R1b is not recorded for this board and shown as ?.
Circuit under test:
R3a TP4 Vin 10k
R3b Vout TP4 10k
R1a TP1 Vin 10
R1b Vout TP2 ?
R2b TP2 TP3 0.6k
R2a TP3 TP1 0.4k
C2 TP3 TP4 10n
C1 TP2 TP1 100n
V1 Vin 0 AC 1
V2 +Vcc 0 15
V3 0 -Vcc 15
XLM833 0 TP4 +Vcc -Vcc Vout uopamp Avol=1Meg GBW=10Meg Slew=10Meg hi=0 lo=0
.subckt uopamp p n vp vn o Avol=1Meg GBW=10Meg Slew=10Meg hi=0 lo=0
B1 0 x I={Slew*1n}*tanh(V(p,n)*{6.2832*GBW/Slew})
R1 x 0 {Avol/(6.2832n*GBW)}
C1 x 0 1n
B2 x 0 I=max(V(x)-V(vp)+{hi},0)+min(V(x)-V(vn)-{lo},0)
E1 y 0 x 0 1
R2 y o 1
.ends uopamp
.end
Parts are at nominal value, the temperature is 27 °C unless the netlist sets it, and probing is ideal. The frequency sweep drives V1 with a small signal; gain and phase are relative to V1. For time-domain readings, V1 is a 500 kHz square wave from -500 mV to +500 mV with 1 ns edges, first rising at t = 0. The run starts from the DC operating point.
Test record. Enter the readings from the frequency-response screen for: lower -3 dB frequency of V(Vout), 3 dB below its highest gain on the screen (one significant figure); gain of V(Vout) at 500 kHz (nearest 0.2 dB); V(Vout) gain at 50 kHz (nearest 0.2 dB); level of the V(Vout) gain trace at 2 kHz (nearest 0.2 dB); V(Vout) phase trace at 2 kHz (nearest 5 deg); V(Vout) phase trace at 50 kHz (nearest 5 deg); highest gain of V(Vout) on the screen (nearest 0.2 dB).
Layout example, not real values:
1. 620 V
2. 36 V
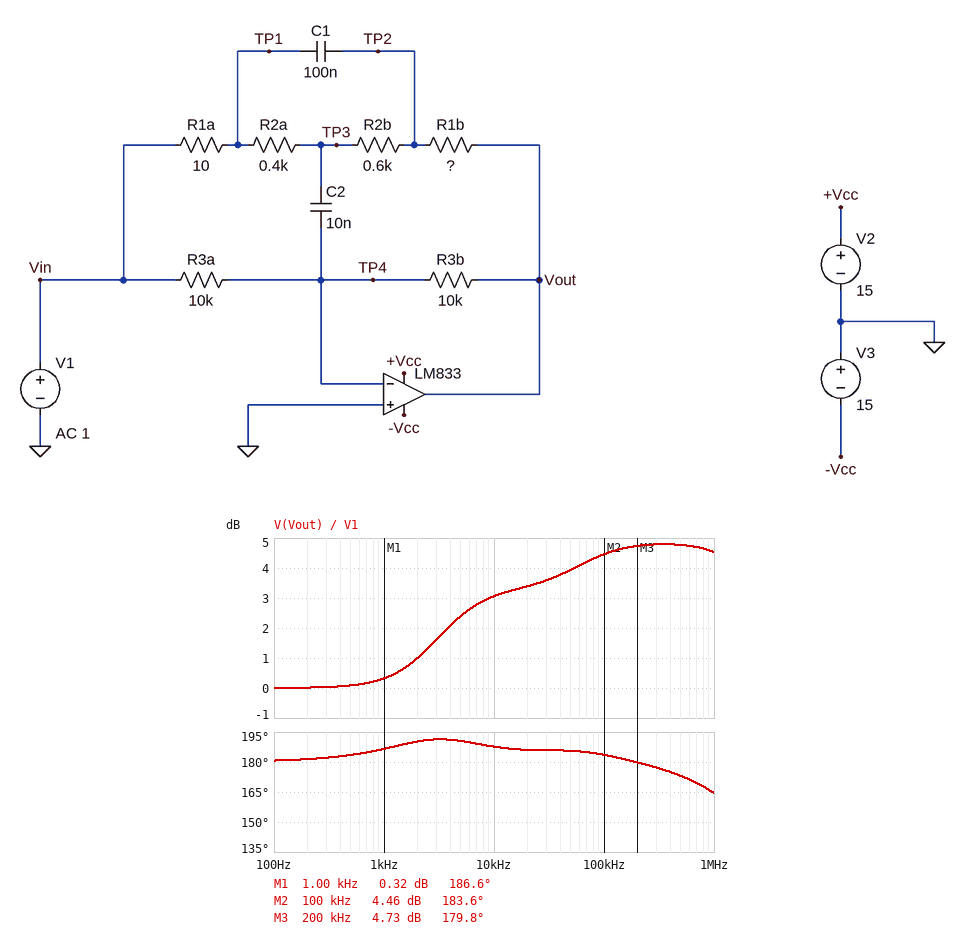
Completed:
1. 3 kHz
2. 4.8 dB
3. 4.0 dB
4. 1.0 dB
5. 190 deg
6. 185 deg
7. 4.8 dB
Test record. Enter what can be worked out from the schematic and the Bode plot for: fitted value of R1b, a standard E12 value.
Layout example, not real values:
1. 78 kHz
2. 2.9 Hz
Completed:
1. 18 Ω
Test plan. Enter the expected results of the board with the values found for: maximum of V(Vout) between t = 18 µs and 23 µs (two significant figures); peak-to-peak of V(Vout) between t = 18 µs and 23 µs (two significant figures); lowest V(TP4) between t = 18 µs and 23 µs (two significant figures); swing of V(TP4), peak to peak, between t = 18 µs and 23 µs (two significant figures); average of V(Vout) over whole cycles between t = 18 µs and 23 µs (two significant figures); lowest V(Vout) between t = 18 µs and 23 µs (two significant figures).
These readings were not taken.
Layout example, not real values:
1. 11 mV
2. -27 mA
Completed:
1. 750 mV
2. 1.8 V
3. -650 mV
4. 1.3 V
5. -140 mV
6. -1.0 V
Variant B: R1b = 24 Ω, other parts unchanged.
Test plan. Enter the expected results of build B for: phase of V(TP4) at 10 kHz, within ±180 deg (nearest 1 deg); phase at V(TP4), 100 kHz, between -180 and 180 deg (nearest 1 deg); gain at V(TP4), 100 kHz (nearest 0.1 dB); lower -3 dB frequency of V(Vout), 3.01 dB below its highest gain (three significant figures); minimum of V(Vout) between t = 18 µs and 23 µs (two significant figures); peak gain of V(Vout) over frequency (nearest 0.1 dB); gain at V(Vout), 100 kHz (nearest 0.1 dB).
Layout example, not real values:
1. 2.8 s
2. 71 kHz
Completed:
1. 101 deg
2. 100 deg
3. -33.3 dB
4. 28.0 kHz
5. -1.3 V
6. 7.1 dB
7. 6.4 dB
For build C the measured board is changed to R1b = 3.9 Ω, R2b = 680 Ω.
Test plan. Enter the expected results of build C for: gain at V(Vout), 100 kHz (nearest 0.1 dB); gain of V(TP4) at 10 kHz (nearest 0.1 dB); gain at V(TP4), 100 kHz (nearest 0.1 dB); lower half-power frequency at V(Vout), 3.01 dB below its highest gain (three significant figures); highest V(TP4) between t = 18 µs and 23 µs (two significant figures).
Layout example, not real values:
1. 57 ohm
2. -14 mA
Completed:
1. -0.5 dB
2. -55.9 dB
3. -40.2 dB
4. 1.79 kHz
5. 330 mV
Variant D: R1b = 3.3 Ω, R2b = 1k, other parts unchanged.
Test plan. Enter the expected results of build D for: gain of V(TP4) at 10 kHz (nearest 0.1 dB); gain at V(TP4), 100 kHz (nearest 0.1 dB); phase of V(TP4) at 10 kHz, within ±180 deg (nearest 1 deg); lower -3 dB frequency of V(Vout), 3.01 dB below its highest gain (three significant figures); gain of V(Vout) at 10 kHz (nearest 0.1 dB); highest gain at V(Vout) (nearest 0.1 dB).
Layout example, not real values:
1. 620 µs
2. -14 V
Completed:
1. -53.1 dB
2. -39.0 dB
3. 96 deg
4. 3.51 kHz
5. 6.9 dB
6. 7.1 dB
